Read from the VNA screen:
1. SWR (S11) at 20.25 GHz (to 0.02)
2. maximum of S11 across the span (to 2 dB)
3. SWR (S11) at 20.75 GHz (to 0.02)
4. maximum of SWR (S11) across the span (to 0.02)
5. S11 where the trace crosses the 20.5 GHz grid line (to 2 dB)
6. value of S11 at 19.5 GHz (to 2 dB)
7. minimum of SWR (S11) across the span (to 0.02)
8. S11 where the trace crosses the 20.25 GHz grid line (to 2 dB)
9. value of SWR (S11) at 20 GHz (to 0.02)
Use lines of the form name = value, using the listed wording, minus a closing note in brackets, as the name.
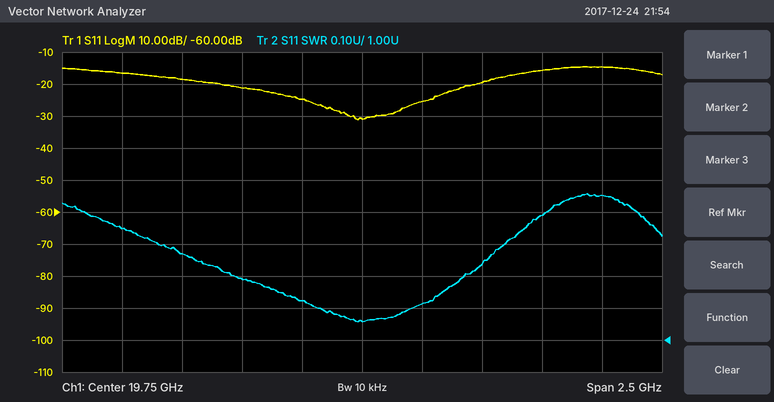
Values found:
SWR (S11) at 20.25 GHz = 1.24
maximum of S11 across the span = -14 dB
SWR (S11) at 20.75 GHz = 1.46
maximum of SWR (S11) across the span = 1.46
S11 where the trace crosses the 20.5 GHz grid line = -16 dB
value of S11 at 19.5 GHz = -24 dB
minimum of SWR (S11) across the span = 1.06
S11 where the trace crosses the 20.25 GHz grid line = -20 dB
value of SWR (S11) at 20 GHz = 1.12
